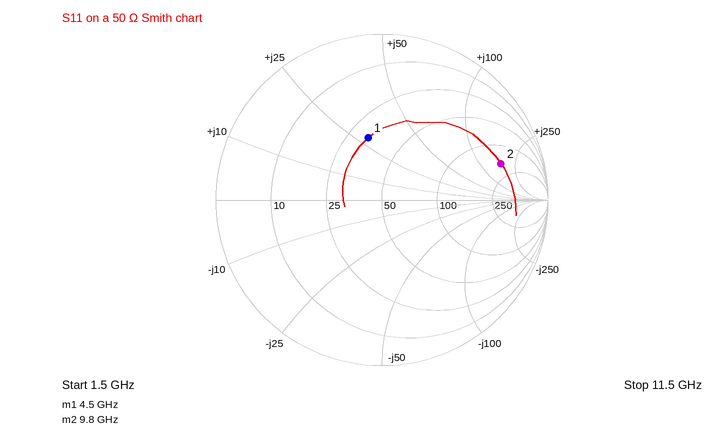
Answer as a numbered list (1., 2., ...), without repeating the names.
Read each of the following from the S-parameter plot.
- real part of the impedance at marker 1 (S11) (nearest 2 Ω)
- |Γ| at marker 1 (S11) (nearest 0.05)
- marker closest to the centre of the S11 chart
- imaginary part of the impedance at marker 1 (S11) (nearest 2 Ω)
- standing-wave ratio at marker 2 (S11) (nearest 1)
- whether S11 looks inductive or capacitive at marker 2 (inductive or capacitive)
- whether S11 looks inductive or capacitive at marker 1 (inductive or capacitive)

1. 32 Ω
2. 0.40
3. marker 1
4. +28 Ω
5. 7
6. inductive
7. inductive
